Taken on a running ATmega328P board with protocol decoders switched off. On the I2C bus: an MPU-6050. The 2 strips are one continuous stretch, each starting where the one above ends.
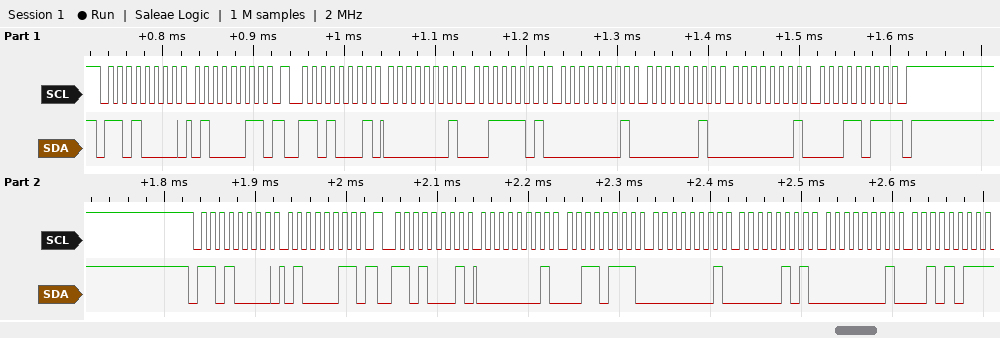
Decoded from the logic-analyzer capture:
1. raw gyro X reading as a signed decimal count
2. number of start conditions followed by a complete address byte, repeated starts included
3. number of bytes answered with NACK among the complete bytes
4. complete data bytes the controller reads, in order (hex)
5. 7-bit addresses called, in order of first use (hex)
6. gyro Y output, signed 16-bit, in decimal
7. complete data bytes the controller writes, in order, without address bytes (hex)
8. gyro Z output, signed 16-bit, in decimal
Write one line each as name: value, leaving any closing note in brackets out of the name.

raw gyro X reading as a signed decimal count: 317
number of start conditions followed by a complete address byte, repeated starts included: 4
number of bytes answered with NACK among the complete bytes: 2
complete data bytes the controller reads, in order: 01 3D 01 02 01 1B 01 37 01 05 01 2B
7-bit addresses called, in order of first use: 0x68
gyro Y output, signed 16-bit, in decimal: 258
complete data bytes the controller writes, in order, without address bytes: 43 43
gyro Z output, signed 16-bit, in decimal: 283
